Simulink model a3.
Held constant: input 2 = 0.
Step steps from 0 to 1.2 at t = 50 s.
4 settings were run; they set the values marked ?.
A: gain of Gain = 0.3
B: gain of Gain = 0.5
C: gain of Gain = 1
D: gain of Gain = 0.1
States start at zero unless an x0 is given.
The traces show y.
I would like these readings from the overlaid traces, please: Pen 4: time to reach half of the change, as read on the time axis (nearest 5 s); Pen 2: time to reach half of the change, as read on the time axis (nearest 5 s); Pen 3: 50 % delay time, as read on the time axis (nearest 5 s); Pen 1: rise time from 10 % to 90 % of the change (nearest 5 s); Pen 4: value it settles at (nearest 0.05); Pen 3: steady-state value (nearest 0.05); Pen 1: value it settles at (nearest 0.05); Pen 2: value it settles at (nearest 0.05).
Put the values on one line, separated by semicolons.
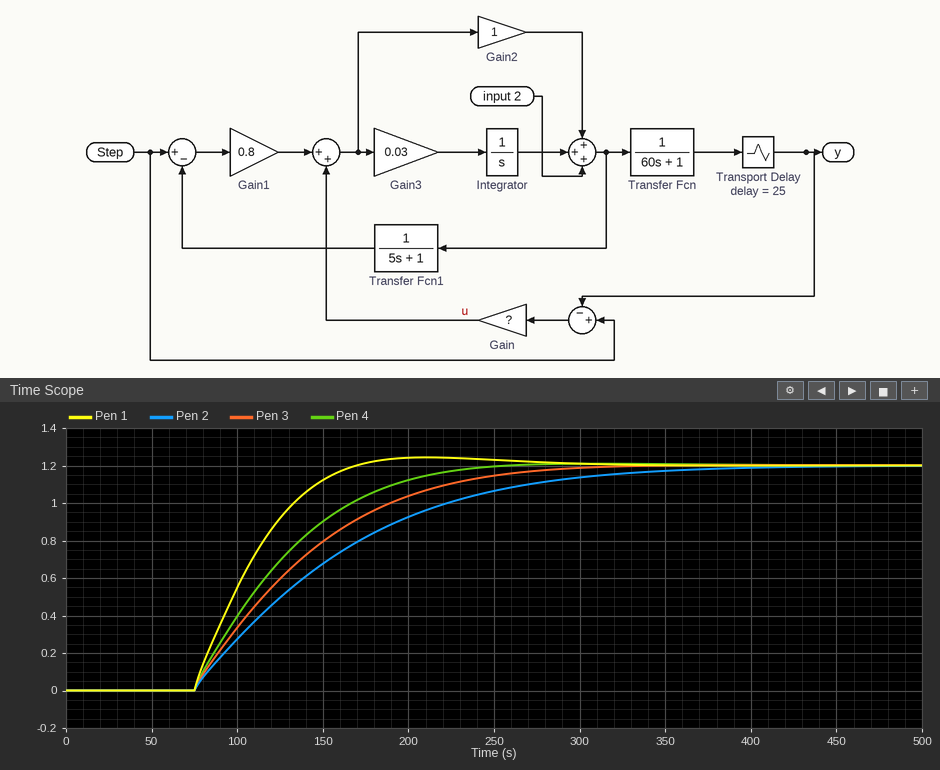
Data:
115 s; 140 s; 125 s; 65 s; 1.20; 1.20; 1.20; 1.20
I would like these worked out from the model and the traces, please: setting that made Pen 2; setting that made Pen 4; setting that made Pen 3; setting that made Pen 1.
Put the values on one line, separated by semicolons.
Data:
D; B; A; C
